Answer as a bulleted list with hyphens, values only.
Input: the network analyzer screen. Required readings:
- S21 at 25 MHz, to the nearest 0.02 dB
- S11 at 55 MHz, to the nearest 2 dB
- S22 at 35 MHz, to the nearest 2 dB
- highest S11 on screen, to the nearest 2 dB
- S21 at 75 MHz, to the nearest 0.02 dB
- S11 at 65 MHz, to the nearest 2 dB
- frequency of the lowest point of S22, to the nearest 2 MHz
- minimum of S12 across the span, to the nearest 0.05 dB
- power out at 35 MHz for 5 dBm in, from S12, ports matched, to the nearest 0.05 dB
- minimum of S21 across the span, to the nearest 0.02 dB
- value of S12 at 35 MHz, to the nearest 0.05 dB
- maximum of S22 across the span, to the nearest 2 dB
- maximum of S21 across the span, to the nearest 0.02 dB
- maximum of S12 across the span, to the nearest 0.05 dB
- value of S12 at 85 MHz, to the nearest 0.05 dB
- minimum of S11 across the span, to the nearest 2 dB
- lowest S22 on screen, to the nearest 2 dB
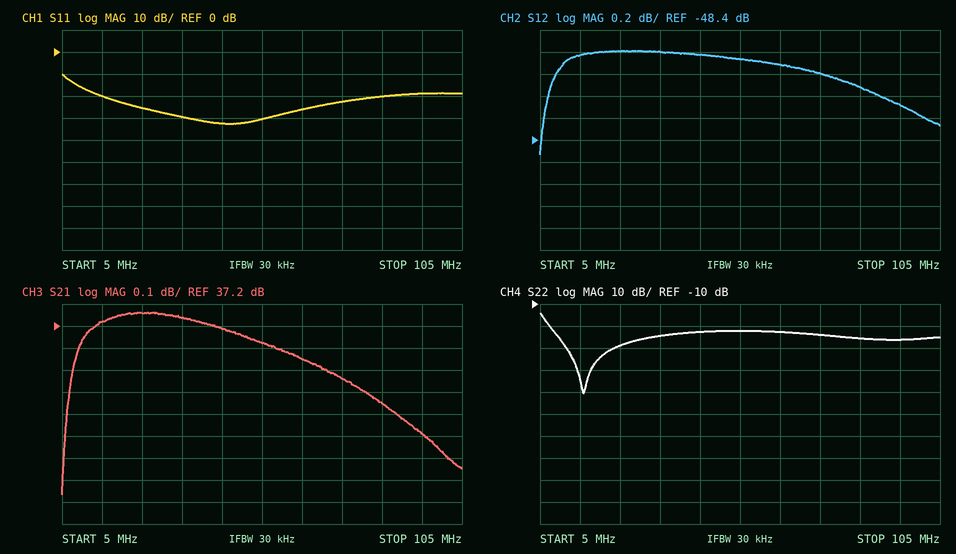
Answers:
- 37.26 dB
- -30 dB
- -24 dB
- -10 dB
- 36.96 dB
- -26 dB
- 16 MHz
- -48.55 dB
- -42.60 dBm
- 36.44 dB
- -47.60 dB
- -14 dB
- 37.26 dB
- -47.60 dB
- -47.90 dB
- -32 dB
- -50 dB
